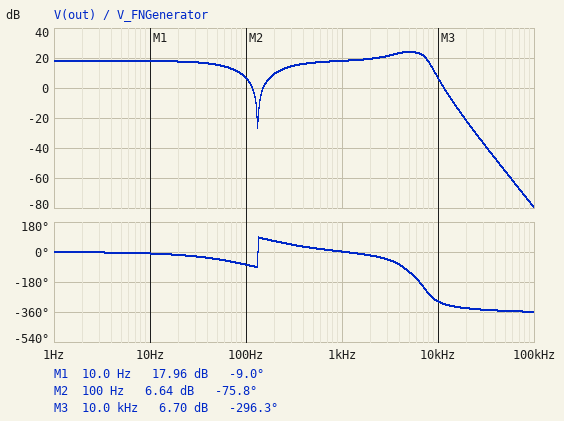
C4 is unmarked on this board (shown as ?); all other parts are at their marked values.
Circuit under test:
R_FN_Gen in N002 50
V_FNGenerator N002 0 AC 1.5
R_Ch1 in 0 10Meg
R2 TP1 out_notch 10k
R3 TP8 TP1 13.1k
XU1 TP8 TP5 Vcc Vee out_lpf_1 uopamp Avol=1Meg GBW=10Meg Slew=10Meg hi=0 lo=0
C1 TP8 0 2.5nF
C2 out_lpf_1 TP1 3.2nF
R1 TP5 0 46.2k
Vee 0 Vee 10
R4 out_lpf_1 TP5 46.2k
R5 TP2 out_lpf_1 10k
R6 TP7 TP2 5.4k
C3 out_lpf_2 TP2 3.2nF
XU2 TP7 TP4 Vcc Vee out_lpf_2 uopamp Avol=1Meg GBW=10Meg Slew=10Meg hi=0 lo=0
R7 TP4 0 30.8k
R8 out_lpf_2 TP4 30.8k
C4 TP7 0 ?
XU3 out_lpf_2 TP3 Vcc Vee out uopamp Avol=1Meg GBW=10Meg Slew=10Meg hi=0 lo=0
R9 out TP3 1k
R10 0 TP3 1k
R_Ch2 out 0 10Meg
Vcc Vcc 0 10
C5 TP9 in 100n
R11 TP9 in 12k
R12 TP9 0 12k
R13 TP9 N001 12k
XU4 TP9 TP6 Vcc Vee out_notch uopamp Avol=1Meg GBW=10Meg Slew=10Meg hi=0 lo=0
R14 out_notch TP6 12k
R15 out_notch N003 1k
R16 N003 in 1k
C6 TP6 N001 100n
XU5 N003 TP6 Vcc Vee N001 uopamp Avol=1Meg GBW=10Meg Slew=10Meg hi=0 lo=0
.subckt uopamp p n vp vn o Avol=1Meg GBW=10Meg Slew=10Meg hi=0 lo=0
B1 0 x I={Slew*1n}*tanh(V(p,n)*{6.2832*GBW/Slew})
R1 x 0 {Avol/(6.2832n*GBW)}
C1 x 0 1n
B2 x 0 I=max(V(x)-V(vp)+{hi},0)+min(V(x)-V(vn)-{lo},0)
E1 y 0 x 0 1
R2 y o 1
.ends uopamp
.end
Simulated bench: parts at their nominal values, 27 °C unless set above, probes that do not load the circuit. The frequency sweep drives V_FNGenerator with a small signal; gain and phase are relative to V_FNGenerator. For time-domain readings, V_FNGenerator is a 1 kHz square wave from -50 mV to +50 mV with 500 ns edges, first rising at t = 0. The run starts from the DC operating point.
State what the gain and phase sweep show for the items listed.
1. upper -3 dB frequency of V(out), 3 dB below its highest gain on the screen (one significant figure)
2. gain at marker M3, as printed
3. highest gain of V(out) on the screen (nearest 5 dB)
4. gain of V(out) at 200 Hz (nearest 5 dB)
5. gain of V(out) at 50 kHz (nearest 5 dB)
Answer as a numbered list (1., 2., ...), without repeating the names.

1. 7 kHz
2. 6.70 dB
3. 25 dB
4. 10 dB
5. -55 dB
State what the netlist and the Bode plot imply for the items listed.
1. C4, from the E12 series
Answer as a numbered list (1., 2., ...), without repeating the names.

1. 2.7 nF
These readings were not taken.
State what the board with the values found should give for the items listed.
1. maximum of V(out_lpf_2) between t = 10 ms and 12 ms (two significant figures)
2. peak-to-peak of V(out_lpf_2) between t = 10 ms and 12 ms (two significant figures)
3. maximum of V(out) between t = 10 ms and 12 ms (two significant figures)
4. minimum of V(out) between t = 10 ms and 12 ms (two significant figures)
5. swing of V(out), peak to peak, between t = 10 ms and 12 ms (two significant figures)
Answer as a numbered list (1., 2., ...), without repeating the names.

1. 470 mV
2. 950 mV
3. 950 mV
4. -950 mV
5. 1.9 V
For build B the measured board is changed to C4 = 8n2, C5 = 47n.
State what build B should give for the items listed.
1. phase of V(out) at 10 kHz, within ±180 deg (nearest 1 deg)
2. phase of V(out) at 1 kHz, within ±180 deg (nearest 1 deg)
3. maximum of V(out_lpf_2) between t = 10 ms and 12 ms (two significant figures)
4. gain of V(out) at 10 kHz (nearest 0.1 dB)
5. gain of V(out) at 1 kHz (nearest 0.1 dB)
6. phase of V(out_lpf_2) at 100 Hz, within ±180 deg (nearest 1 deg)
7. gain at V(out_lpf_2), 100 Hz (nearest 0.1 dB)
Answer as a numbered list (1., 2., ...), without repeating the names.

1. 82 deg
2. -11 deg
3. 230 mV
4. -10.5 dB
5. 16.0 dB
6. -69 deg
7. 4.7 dB
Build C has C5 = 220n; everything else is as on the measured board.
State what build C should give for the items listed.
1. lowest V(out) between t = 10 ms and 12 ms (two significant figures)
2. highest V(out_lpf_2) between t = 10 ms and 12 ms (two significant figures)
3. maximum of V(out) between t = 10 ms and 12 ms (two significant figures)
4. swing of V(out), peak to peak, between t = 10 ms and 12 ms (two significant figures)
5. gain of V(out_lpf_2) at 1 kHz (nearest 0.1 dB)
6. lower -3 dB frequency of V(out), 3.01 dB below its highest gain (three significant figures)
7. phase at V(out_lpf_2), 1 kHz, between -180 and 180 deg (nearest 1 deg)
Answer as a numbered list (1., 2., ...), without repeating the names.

1. -900 mV
2. 460 mV
3. 920 mV
4. 1.8 V
5. 12.3 dB
6. 2.82 kHz
7. -6 deg
